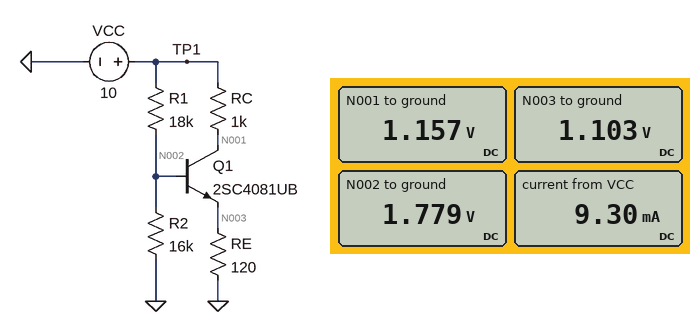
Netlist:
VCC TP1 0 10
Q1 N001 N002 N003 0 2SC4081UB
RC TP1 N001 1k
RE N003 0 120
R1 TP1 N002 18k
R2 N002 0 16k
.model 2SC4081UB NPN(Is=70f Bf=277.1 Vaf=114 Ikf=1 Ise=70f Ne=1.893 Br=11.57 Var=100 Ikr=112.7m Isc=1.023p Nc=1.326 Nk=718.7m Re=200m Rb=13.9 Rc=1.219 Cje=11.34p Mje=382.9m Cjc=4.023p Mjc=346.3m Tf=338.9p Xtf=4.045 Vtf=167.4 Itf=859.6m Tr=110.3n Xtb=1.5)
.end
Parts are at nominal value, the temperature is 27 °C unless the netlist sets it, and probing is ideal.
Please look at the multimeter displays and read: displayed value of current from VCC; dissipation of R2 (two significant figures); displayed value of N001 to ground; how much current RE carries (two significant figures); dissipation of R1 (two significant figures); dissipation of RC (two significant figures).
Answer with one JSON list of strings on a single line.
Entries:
["9.30 mA", "200 µW", "1.157 V", "9.2 mA", "3.8 mW", "78 mW"]
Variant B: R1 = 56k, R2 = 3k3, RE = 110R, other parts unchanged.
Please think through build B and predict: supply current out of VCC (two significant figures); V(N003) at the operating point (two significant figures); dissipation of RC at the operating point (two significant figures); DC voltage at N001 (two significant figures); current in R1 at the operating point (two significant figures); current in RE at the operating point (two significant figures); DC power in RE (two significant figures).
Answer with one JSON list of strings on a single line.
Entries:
["270 µA", "11 mV", "11 µW", "9.9 V", "170 µA", "100 µA", "1.2 µW"]
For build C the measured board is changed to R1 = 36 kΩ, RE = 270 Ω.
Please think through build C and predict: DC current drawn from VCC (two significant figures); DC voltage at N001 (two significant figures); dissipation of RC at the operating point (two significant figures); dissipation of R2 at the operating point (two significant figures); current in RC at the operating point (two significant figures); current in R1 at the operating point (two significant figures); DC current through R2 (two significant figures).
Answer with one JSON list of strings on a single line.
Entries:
["7.9 mA", "2.3 V", "59 mW", "470 µW", "7.7 mA", "200 µA", "170 µA"]
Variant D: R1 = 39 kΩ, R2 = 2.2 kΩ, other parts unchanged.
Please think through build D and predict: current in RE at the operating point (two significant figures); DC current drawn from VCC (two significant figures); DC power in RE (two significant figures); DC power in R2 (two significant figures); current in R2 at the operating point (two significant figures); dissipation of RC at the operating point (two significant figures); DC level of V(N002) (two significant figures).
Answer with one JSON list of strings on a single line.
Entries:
["54 µA", "300 µA", "350 nW", "130 µW", "240 µA", "2.9 µW", "530 mV"]
